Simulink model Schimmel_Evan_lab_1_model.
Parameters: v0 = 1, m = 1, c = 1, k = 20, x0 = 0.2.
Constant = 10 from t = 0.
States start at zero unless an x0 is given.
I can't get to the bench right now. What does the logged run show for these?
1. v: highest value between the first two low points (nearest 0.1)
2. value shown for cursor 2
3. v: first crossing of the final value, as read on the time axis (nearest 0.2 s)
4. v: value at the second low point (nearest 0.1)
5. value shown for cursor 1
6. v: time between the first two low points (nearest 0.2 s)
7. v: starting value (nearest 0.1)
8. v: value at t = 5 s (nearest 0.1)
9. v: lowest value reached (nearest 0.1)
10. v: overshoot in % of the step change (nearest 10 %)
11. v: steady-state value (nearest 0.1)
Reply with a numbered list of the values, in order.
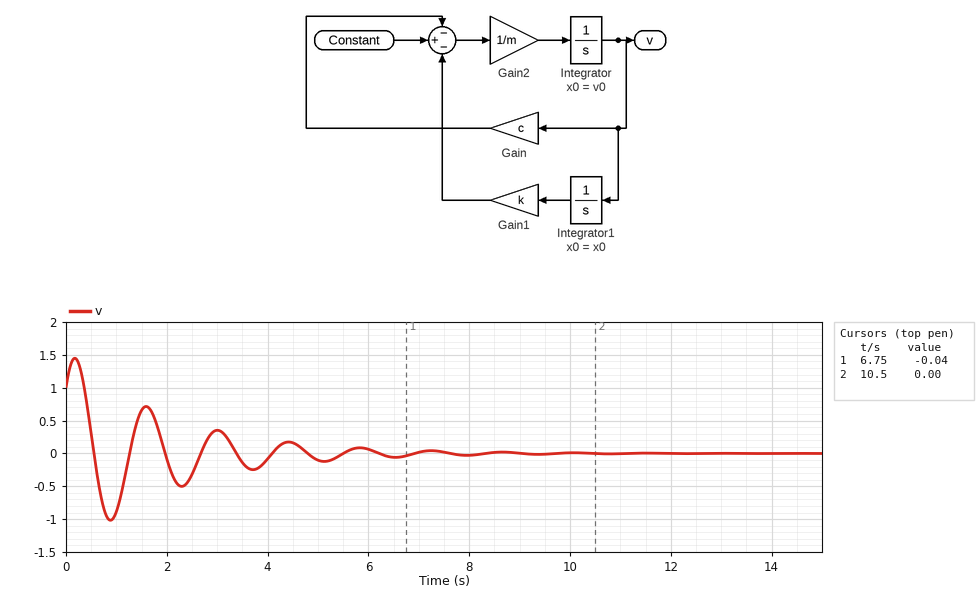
1. 0.7
2. 0.00
3. 0.6 s
4. -0.5
5. -0.04
6. 1.4 s
7. 1.0
8. -0.1
9. -1.0
10. 100 %
11. 0.0
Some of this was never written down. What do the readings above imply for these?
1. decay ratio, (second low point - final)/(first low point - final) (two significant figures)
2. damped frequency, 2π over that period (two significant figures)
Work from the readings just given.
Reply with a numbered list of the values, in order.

1. 0.50
2. 4.5 rad/s
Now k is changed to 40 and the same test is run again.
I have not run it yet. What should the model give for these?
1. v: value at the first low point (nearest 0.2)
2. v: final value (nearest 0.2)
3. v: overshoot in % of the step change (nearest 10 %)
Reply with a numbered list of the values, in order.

1. -0.8
2. 0.0
3. 80 %
